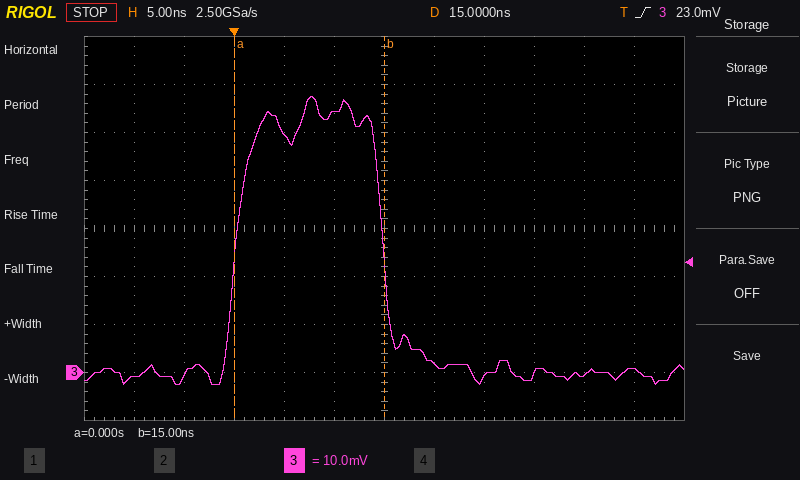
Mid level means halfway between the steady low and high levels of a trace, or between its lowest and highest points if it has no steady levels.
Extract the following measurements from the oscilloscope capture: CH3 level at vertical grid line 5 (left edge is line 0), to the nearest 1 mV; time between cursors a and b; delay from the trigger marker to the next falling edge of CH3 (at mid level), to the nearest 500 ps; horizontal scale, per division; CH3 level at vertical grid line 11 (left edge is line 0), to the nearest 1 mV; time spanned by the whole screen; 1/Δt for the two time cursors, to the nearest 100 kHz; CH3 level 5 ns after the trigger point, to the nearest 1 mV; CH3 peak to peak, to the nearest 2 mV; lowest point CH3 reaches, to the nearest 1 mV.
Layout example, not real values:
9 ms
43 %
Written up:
54 mV
15.0 ns
15.0 ns
5 ns
1 mV
60 ns
66.7 MHz
50 mV
60 mV
-2 mV
